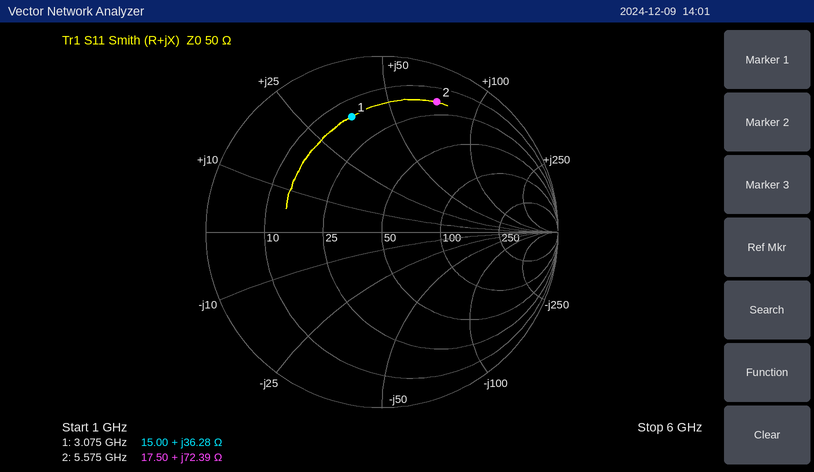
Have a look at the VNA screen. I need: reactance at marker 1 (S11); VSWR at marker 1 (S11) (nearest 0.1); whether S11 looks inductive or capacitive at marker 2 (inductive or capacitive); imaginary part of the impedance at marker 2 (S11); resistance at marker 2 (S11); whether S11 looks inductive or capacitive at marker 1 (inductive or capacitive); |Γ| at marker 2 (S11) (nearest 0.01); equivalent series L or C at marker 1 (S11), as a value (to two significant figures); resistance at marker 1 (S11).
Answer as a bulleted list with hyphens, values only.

- +36.28 Ω
- 5.2
- inductive
- +72.39 Ω
- 17.50 Ω
- inductive
- 0.80
- 1.9 nH
- 15.00 Ω
